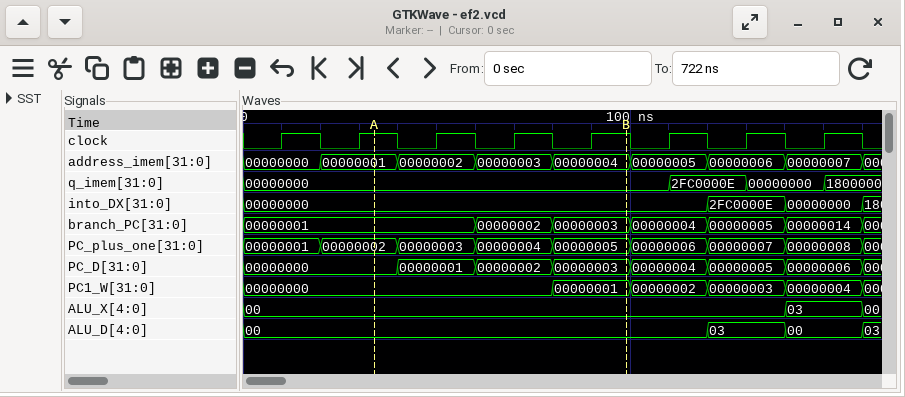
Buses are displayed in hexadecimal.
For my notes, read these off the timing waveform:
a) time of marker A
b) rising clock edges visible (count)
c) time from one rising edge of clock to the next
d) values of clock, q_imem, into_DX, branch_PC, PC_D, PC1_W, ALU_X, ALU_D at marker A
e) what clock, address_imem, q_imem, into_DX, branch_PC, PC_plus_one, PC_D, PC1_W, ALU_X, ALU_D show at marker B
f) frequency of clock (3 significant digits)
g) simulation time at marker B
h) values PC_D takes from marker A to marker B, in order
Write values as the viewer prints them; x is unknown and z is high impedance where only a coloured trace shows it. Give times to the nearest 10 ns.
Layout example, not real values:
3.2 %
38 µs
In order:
30 ns
8
20 ns
clock=1, q_imem=00000000, into_DX=00000000, branch_PC=00000001, PC_D=00000000, PC1_W=00000000, ALU_X=00, ALU_D=00
clock=1, address_imem=00000004, q_imem=00000000, into_DX=00000000, branch_PC=00000003, PC_plus_one=00000005, PC_D=00000003, PC1_W=00000001, ALU_X=00, ALU_D=00
50.0 MHz
100 ns
00000000, 00000001, 00000002, 00000003
